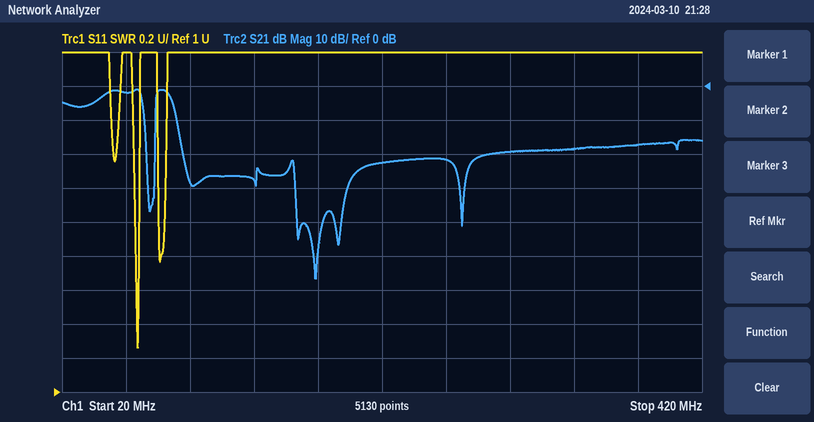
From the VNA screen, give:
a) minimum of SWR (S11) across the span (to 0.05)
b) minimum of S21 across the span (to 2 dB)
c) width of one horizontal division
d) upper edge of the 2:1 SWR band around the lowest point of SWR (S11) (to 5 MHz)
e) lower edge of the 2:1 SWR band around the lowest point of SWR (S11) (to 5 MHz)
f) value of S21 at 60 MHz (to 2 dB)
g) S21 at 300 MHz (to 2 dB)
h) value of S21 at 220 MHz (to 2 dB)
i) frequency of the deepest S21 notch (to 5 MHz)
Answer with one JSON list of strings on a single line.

["1.25", "-56 dB", "40 MHz", "70 MHz", "65 MHz", "-2 dB", "-20 dB", "-22 dB", "180 MHz"]
